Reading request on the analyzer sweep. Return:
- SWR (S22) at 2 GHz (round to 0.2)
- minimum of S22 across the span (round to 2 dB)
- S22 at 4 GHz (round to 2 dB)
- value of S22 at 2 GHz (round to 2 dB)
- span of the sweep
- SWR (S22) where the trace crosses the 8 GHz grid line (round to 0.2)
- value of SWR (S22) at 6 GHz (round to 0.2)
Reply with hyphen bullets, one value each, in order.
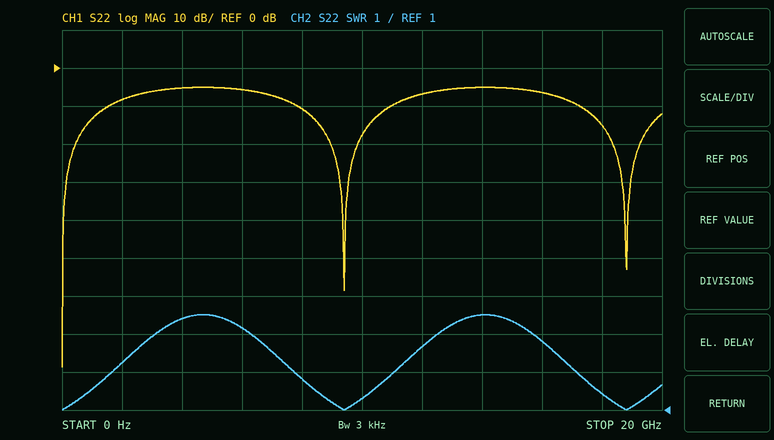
- 2.2
- -78 dB
- -6 dB
- -8 dB
- 20 GHz
- 1.8
- 3.2
